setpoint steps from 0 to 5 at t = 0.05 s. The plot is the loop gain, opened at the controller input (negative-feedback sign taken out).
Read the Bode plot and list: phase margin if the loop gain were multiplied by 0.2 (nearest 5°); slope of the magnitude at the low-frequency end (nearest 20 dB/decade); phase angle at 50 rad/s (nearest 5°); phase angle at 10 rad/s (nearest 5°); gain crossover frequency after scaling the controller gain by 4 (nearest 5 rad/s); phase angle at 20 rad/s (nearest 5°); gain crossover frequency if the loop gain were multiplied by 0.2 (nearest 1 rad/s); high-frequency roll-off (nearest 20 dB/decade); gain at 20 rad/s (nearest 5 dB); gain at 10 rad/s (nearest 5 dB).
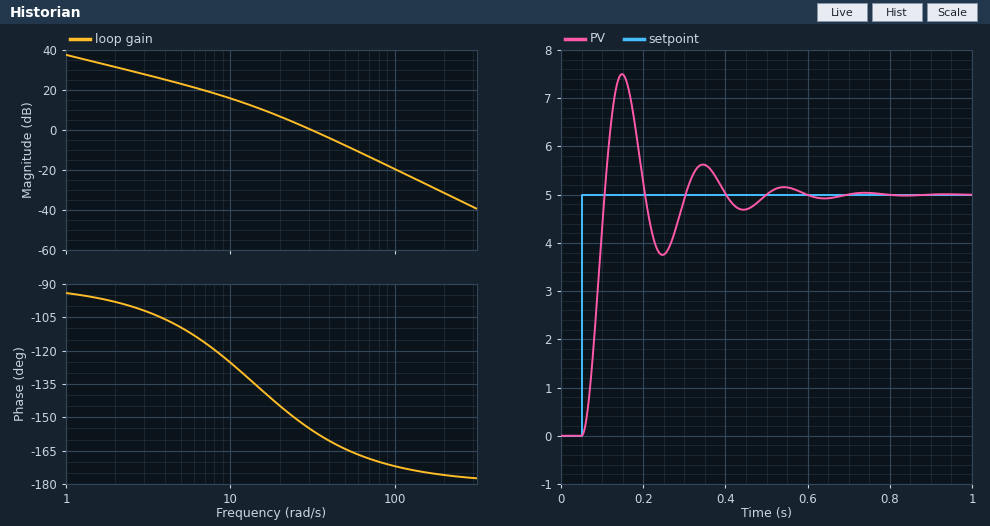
50°
-20 dB/decade
-165°
-125°
65 rad/s
-145°
12 rad/s
-40 dB/decade
5 dB
15 dB
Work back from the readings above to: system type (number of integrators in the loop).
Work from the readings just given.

1
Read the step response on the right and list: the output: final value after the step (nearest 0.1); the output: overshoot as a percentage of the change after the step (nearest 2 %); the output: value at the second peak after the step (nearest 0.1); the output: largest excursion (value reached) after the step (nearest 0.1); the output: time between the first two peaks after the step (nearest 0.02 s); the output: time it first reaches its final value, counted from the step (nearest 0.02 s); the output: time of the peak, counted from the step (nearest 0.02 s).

5.0
50 %
5.6
7.5
0.20 s
0.06 s
0.10 s
